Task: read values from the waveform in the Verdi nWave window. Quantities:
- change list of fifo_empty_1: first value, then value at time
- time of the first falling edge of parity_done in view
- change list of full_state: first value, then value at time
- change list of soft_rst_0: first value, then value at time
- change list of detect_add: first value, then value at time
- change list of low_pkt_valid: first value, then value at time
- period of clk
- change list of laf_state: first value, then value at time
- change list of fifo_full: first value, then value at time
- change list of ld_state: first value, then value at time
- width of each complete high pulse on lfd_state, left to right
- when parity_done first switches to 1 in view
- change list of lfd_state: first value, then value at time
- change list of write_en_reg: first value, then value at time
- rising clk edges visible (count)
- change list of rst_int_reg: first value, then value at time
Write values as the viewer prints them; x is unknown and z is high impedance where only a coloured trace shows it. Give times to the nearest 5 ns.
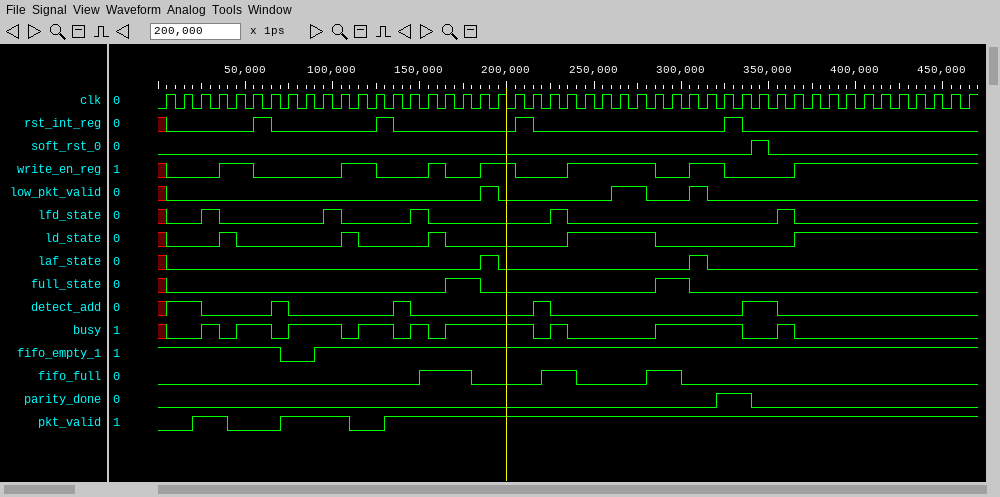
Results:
1, 0 at 70 ns, 1 at 90 ns
340 ns
x, 0 at 5 ns, 1 at 165 ns, 0 at 185 ns, 1 at 285 ns, 0 at 305 ns
0, 1 at 340 ns, 0 at 350 ns
x, 1 at 5 ns, 0 at 25 ns, 1 at 65 ns, 0 at 75 ns, 1 at 135 ns, 0 at 145 ns, 1 at 215 ns, 0 at 225 ns, 1 at 335 ns, 0 at 355 ns
x, 0 at 5 ns, 1 at 185 ns, 0 at 195 ns, 1 at 260 ns, 0 at 280 ns, 1 at 305 ns, 0 at 315 ns
10 ns
x, 0 at 5 ns, 1 at 185 ns, 0 at 195 ns, 1 at 305 ns, 0 at 315 ns
0, 1 at 150 ns, 0 at 180 ns, 1 at 220 ns, 0 at 240 ns, 1 at 280 ns, 0 at 300 ns
x, 0 at 5 ns, 1 at 35 ns, 0 at 45 ns, 1 at 105 ns, 0 at 115 ns, 1 at 155 ns, 0 at 165 ns, 1 at 235 ns, 0 at 285 ns, 1 at 365 ns
10 ns, 10 ns, 10 ns, 10 ns, 10 ns
320 ns
x, 0 at 5 ns, 1 at 25 ns, 0 at 35 ns, 1 at 95 ns, 0 at 105 ns, 1 at 145 ns, 0 at 155 ns, 1 at 225 ns, 0 at 235 ns, 1 at 355 ns, 0 at 365 ns
x, 0 at 5 ns, 1 at 35 ns, 0 at 55 ns, 1 at 105 ns, 0 at 125 ns, 1 at 155 ns, 0 at 165 ns, 1 at 185 ns, 0 at 205 ns, 1 at 235 ns, 0 at 285 ns, 1 at 305 ns, 0 at 325 ns, 1 at 365 ns
47
x, 0 at 5 ns, 1 at 55 ns, 0 at 65 ns, 1 at 125 ns, 0 at 135 ns, 1 at 205 ns, 0 at 215 ns, 1 at 325 ns, 0 at 335 ns
